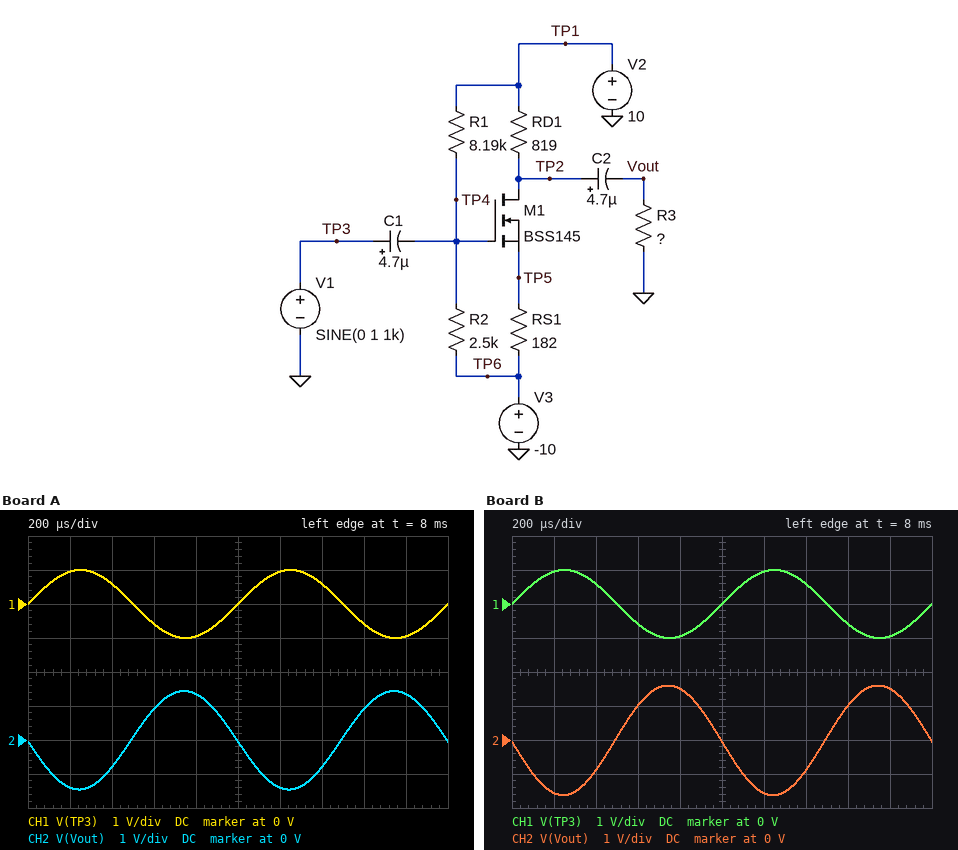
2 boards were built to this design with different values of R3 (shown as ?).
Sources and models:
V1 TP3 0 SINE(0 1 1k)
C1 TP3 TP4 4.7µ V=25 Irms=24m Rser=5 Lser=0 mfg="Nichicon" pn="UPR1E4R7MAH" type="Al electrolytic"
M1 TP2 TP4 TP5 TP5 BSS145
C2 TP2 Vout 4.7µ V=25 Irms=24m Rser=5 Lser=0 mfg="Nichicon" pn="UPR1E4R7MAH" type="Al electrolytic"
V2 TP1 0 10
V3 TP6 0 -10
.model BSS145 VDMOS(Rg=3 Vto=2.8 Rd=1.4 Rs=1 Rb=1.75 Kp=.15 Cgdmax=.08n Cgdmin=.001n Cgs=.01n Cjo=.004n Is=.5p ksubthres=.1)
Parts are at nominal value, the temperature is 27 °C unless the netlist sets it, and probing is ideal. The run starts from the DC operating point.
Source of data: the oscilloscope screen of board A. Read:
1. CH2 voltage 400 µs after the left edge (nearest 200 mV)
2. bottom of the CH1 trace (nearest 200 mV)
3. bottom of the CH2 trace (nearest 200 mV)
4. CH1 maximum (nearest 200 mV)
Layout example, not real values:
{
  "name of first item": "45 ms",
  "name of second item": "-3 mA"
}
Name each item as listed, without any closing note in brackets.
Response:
{
  "CH2 voltage 400 µs after the left edge": "-800 mV",
  "bottom of the CH1 trace": "-1.0 V",
  "bottom of the CH2 trace": "-1.4 V",
  "CH1 maximum": "1.0 V"
}
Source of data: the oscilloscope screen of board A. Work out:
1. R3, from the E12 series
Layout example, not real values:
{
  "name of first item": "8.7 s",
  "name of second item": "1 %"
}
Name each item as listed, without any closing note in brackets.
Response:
{
  "R3, from the E12 series": "470 Ω"
}
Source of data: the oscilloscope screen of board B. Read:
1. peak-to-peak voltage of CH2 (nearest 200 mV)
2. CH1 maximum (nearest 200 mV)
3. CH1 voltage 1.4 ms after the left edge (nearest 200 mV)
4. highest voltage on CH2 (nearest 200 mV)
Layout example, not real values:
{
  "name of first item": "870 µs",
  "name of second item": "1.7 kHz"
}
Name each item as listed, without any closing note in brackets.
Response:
{
  "peak-to-peak voltage of CH2": "3.2 V",
  "CH1 maximum": "1.0 V",
  "CH1 voltage 1.4 ms after the left edge": "600 mV",
  "highest voltage on CH2": "1.6 V"
}
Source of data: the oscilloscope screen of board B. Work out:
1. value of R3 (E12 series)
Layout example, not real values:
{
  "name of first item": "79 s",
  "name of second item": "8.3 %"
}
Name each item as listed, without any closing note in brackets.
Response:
{
  "value of R3": "560 Ω"
}
